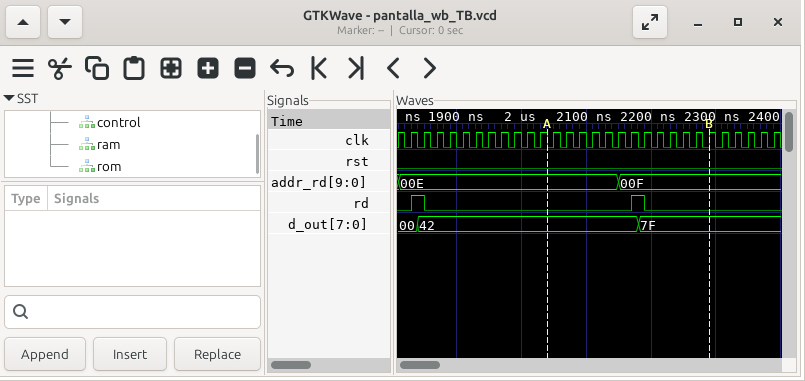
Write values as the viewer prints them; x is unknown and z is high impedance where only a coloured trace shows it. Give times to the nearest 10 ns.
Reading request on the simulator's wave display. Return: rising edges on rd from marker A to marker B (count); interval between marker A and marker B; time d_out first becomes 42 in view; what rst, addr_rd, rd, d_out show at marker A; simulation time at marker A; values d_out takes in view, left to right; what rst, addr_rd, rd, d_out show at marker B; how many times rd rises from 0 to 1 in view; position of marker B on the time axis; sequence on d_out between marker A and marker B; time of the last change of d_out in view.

1
250 ns
1840 ns
rst=0, addr_rd=00E, rd=0, d_out=42
2040 ns
00, 42, 7F
rst=0, addr_rd=00F, rd=0, d_out=7F
2
2290 ns
42, 7F
2180 ns
